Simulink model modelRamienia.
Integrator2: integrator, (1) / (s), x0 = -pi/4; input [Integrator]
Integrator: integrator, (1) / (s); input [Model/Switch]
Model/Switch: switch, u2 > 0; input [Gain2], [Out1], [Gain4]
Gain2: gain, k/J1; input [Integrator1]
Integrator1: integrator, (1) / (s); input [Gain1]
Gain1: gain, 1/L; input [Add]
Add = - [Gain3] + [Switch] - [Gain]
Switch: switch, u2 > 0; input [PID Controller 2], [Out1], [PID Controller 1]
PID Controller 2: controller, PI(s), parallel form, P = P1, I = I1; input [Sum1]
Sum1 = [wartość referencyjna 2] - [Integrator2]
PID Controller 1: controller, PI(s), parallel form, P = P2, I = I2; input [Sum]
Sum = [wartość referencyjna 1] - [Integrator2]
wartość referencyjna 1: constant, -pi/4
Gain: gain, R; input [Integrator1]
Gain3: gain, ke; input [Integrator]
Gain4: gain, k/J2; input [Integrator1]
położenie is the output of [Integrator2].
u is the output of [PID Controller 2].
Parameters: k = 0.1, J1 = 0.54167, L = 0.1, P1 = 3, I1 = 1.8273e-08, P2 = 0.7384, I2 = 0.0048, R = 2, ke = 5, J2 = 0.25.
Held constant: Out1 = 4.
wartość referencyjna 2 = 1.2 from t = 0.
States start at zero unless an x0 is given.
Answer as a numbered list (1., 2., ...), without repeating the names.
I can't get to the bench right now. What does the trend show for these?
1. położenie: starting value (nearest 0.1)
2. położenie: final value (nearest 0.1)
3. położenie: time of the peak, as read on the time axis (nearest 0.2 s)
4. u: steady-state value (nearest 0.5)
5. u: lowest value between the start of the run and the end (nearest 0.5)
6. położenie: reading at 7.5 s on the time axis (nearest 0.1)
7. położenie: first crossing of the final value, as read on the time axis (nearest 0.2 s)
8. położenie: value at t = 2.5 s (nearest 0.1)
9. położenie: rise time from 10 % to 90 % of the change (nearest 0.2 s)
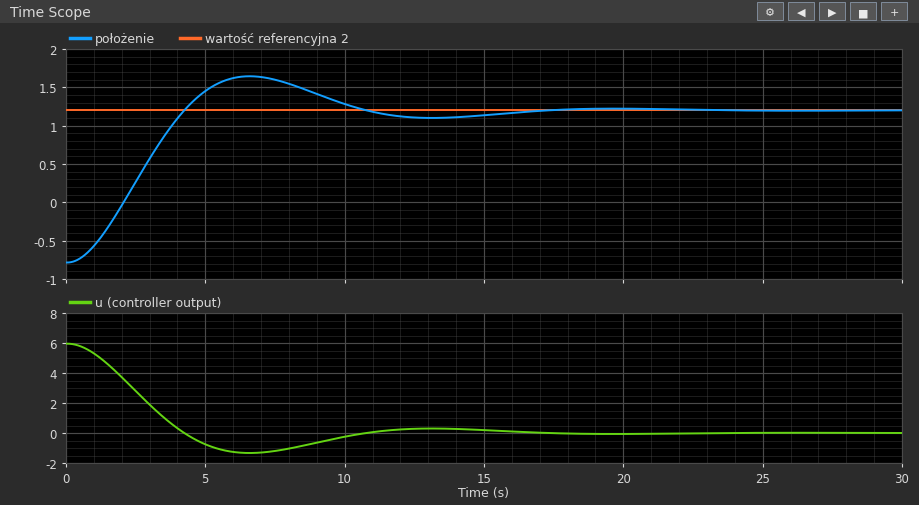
1. -0.8
2. 1.2
3. 6.6 s
4. 0.0
5. -1.5
6. 1.6
7. 4.2 s
8. 0.3
9. 2.8 s
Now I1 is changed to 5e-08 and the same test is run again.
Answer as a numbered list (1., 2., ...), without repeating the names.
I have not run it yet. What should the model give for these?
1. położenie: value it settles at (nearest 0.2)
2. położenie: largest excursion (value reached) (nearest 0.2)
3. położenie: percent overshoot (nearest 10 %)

1. 1.2
2. 1.6
3. 20 %
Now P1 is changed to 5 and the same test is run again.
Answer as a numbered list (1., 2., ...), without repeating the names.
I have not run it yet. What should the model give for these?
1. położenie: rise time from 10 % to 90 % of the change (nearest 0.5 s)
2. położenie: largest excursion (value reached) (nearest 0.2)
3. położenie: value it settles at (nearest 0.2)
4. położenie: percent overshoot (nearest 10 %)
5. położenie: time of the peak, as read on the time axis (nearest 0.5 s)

1. 2.0 s
2. 1.8
3. 1.2
4. 30 %
5. 5.0 s
